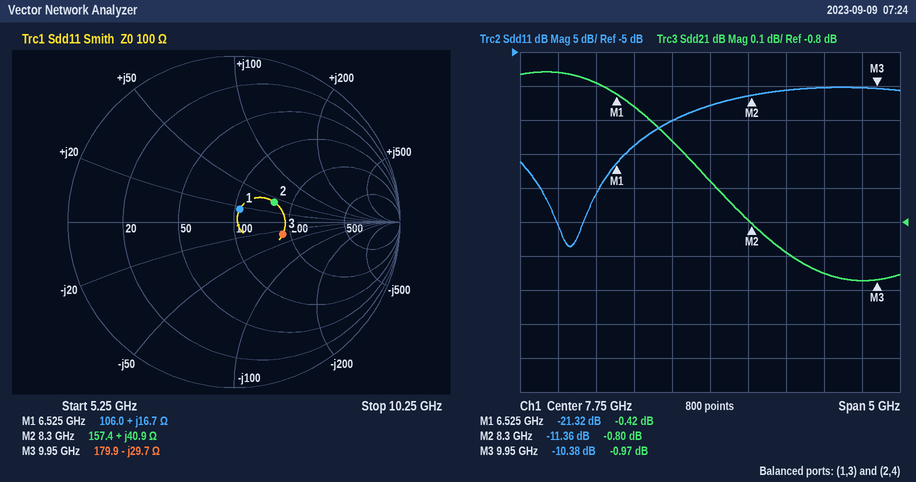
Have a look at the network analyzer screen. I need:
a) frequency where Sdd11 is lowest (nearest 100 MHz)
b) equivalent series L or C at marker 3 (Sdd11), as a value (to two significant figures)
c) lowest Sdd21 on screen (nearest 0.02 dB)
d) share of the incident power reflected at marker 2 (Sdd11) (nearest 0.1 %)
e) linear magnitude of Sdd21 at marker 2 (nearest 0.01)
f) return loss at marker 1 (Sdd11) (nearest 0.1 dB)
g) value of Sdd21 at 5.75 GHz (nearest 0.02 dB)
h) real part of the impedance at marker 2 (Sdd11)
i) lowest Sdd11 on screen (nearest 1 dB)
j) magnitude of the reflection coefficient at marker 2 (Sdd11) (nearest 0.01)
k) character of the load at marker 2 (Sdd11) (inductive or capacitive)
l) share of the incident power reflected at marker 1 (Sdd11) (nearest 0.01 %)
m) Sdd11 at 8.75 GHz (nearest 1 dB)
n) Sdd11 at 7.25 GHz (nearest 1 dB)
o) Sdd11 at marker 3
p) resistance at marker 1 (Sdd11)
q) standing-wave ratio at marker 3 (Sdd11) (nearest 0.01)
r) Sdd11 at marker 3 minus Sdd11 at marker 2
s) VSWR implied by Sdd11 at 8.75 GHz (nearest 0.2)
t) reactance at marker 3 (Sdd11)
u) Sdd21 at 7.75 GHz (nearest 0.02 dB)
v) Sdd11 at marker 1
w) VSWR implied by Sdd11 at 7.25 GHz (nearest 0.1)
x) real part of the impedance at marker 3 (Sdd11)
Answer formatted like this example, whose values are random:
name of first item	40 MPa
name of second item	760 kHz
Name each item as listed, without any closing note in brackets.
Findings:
frequency where Sdd11 is lowest	5.9 GHz
equivalent series L or C at marker 3 (Sdd11), as a value	540 fF
lowest Sdd21 on screen	-0.98 dB
share of the incident power reflected at marker 2 (Sdd11)	7.3 %
linear magnitude of Sdd21 at marker 2	0.91
return loss at marker 1 (Sdd11)	21.3 dB
value of Sdd21 at 5.75 GHz	-0.36 dB
real part of the impedance at marker 2	157.4 Ω
lowest Sdd11 on screen	-34 dB
magnitude of the reflection coefficient at marker 2 (Sdd11)	0.27
character of the load at marker 2 (Sdd11)	inductive
share of the incident power reflected at marker 1 (Sdd11)	0.74 %
Sdd11 at 8.75 GHz	-11 dB
Sdd11 at 7.25 GHz	-15 dB
Sdd11 at marker 3	-10.38 dB
resistance at marker 1	106.0 Ω
standing-wave ratio at marker 3 (Sdd11)	1.87
Sdd11 at marker 3 minus Sdd11 at marker 2	0.98 dB
VSWR implied by Sdd11 at 8.75 GHz	1.8
reactance at marker 3	-29.7 Ω
Sdd21 at 7.75 GHz	-0.68 dB
Sdd11 at marker 1	-21.32 dB
VSWR implied by Sdd11 at 7.25 GHz	1.4
real part of the impedance at marker 3	179.9 Ω
